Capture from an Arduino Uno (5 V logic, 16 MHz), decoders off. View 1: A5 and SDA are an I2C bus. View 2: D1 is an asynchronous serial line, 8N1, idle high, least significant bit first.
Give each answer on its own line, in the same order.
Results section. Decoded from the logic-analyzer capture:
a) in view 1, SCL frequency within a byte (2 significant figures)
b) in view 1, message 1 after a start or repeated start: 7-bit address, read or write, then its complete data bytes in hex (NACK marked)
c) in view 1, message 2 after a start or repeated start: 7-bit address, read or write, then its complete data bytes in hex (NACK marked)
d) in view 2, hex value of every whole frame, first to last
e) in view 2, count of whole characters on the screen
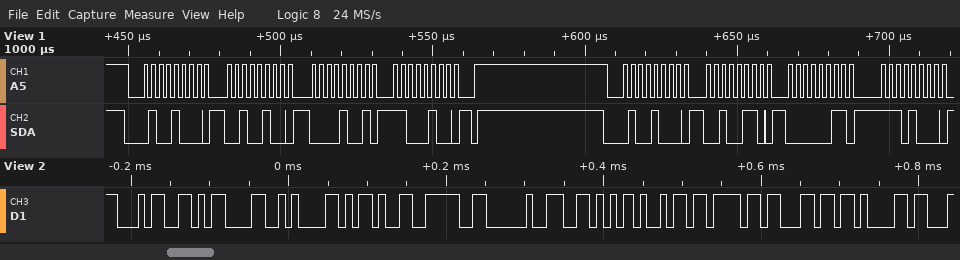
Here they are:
400 kHz
0x24 write: 24 09 C4
0x24 write: 26 03 E8
34 0D 0A 2D 3E 20 56 69 6F 6C 61
11
